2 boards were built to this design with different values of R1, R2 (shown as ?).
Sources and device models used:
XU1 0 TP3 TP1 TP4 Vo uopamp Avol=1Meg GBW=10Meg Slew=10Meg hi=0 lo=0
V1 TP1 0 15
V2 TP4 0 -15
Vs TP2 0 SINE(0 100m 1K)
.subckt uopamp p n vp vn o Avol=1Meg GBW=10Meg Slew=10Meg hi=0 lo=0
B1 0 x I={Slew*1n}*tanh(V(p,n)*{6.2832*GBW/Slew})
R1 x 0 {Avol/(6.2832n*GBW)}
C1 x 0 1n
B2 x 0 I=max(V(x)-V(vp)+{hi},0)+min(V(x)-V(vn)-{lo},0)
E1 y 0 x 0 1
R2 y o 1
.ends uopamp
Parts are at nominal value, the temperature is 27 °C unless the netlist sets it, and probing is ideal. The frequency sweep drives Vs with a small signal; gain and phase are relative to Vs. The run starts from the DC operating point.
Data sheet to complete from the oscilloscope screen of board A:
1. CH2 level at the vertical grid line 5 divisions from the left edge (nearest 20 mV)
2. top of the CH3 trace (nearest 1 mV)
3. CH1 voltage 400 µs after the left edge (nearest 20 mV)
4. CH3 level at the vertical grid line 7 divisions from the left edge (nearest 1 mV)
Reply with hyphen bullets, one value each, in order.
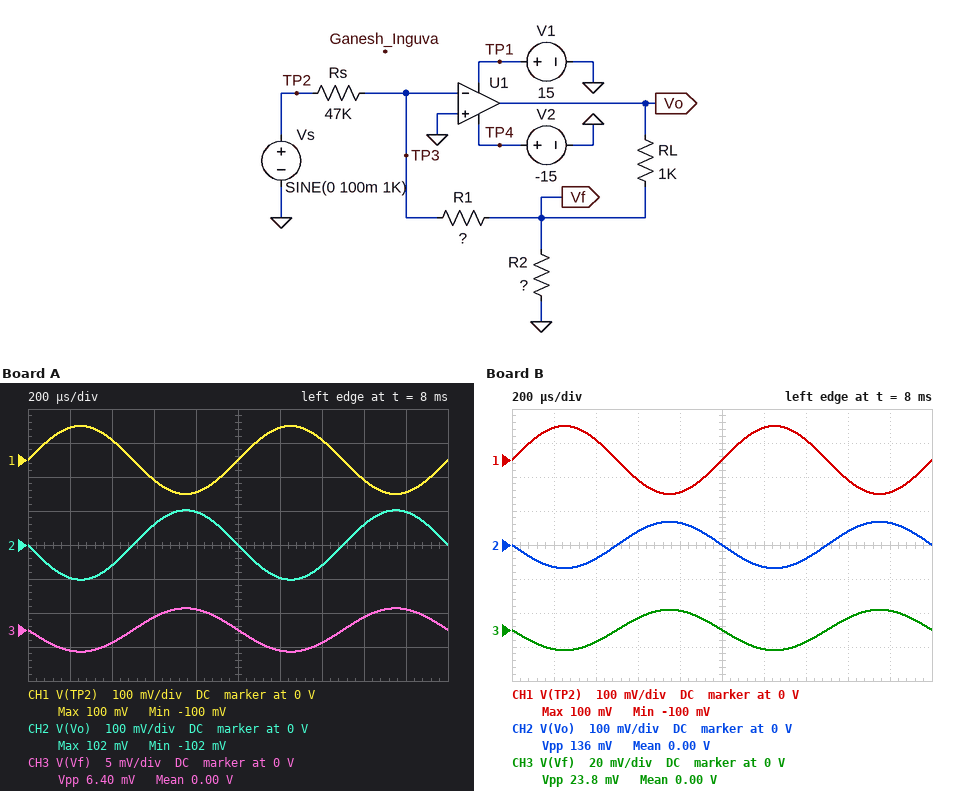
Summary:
- 0 V
- 3 mV
- 60 mV
- -2 mV
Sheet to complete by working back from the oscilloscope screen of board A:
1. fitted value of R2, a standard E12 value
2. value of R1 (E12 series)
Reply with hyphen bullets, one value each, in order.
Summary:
- 33 Ω
- 1.5 kΩ
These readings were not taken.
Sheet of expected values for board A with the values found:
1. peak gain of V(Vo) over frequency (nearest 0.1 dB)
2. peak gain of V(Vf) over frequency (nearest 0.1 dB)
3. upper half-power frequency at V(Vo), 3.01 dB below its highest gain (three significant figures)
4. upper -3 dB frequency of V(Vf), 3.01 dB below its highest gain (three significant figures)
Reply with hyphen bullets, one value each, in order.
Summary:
- 0.2 dB
- -29.9 dB
- 309 kHz
- 309 kHz
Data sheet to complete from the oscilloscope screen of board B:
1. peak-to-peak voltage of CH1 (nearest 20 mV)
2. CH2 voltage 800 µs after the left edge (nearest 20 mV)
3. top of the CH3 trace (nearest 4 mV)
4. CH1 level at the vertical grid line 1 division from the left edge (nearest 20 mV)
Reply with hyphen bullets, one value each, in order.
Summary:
- 200 mV
- 60 mV
- 12 mV
- 100 mV
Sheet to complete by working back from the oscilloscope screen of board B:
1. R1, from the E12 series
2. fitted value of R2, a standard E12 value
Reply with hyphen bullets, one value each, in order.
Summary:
- 5.6 kΩ
- 220 Ω
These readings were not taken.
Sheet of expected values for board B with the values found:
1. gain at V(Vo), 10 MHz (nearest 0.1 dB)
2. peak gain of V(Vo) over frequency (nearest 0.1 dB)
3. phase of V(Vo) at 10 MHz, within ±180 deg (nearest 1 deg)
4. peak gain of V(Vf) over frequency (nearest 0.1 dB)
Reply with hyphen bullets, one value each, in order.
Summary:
- -19.3 dB
- -3.3 dB
- 99 deg
- -18.5 dB
